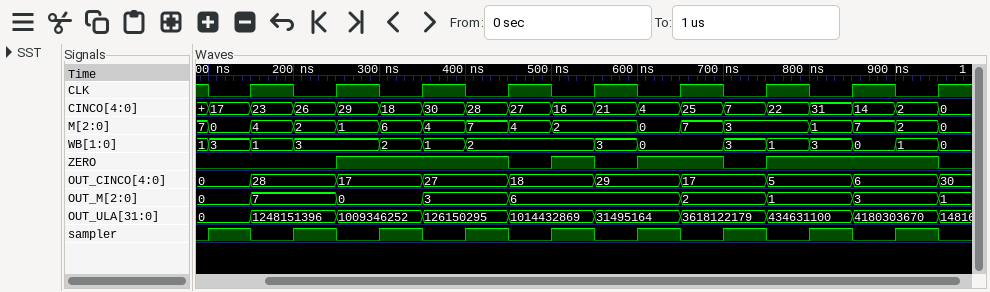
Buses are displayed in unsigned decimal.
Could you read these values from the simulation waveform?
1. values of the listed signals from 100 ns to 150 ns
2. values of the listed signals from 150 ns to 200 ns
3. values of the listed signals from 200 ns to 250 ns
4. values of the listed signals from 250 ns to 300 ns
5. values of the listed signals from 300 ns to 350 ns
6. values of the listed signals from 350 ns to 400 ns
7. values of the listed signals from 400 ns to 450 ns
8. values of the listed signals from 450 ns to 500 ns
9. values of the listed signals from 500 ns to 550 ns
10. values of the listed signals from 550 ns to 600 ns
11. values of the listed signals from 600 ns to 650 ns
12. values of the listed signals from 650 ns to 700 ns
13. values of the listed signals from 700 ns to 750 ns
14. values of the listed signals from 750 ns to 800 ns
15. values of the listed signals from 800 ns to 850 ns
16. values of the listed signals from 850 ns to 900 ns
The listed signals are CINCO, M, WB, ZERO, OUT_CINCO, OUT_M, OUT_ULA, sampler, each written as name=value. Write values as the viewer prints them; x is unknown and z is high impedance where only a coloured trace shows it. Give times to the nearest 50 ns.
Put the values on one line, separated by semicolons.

CINCO=17, M=0, WB=3, ZERO=0, OUT_CINCO=0, OUT_M=0, OUT_ULA=0, sampler=1; CINCO=23, M=4, WB=1, ZERO=0, OUT_CINCO=28, OUT_M=7, OUT_ULA=1248151396, sampler=0; CINCO=26, M=2, WB=3, ZERO=0, OUT_CINCO=28, OUT_M=7, OUT_ULA=1248151396, sampler=1; CINCO=29, M=1, WB=3, ZERO=1, OUT_CINCO=17, OUT_M=0, OUT_ULA=1009346252, sampler=0; CINCO=18, M=6, WB=2, ZERO=1, OUT_CINCO=17, OUT_M=0, OUT_ULA=1009346252, sampler=1; CINCO=30, M=4, WB=1, ZERO=1, OUT_CINCO=27, OUT_M=3, OUT_ULA=126150295, sampler=0; CINCO=28, M=7, WB=2, ZERO=1, OUT_CINCO=27, OUT_M=3, OUT_ULA=126150295, sampler=1; CINCO=27, M=4, WB=2, ZERO=0, OUT_CINCO=18, OUT_M=6, OUT_ULA=1014432869, sampler=0; CINCO=16, M=2, WB=2, ZERO=1, OUT_CINCO=18, OUT_M=6, OUT_ULA=1014432869, sampler=1; CINCO=21, M=2, WB=3, ZERO=0, OUT_CINCO=29, OUT_M=6, OUT_ULA=31495164, sampler=0; CINCO=4, M=0, WB=0, ZERO=1, OUT_CINCO=29, OUT_M=6, OUT_ULA=31495164, sampler=1; CINCO=25, M=7, WB=0, ZERO=1, OUT_CINCO=17, OUT_M=2, OUT_ULA=3618122179, sampler=0; CINCO=7, M=3, WB=3, ZERO=0, OUT_CINCO=17, OUT_M=2, OUT_ULA=3618122179, sampler=1; CINCO=22, M=3, WB=1, ZERO=1, OUT_CINCO=5, OUT_M=1, OUT_ULA=434631100, sampler=0; CINCO=31, M=1, WB=3, ZERO=1, OUT_CINCO=5, OUT_M=1, OUT_ULA=434631100, sampler=1; CINCO=14, M=7, WB=0, ZERO=1, OUT_CINCO=6, OUT_M=3, OUT_ULA=4180303670, sampler=0
